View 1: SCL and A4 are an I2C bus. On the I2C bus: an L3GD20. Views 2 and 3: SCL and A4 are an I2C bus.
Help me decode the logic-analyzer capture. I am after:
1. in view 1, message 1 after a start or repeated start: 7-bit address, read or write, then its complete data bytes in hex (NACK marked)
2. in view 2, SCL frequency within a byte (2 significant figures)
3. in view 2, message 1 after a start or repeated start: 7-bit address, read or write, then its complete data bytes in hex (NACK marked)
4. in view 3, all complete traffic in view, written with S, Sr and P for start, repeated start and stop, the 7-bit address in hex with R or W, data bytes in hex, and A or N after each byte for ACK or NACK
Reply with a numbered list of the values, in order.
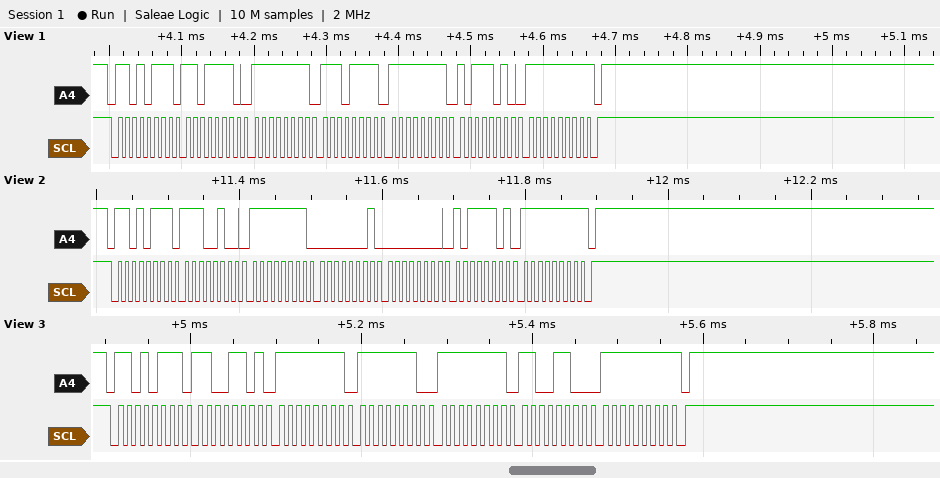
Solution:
1. 0x6B read: DE FF EF FF BA FF NACK
2. 100 kHz
3. 0x6B read: E4 FF 01 00 BD FF NACK
4. S 6BR A CD A FF A FE A FF A CC A FF N P
